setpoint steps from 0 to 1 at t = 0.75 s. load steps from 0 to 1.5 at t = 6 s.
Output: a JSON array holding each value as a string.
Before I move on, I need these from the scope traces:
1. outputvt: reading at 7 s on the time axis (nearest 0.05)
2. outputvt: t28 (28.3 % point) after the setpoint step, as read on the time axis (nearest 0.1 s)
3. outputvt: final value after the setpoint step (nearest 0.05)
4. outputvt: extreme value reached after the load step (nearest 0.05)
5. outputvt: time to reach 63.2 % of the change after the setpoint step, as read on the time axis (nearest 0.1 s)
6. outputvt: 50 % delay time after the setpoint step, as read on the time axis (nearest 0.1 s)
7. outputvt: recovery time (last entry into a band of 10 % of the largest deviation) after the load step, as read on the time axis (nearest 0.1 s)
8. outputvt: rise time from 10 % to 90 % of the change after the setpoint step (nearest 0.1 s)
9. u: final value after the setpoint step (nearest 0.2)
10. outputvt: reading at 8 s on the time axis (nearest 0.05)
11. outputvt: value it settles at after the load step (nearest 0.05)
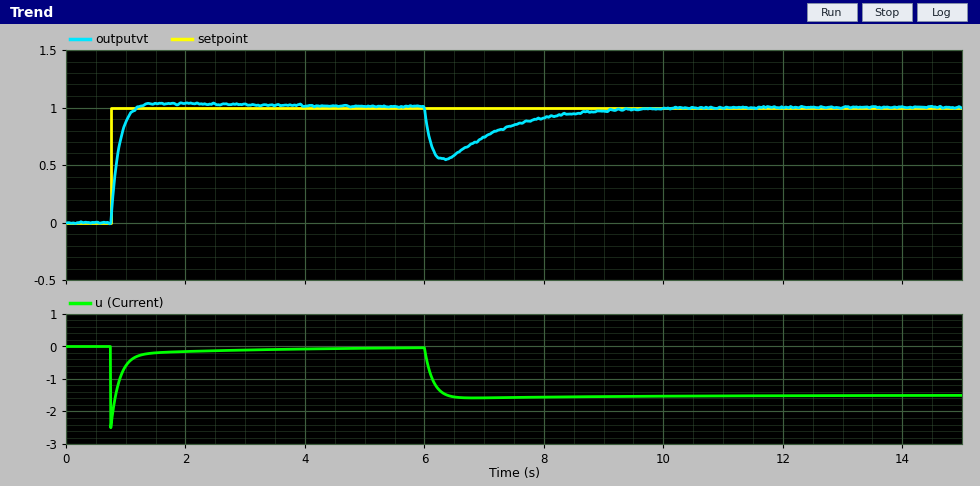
["0.75", "0.8 s", "1.00", "0.55", "0.9 s", "0.8 s", "8.6 s", "0.3 s", "0.0", "0.90", "1.00"]
